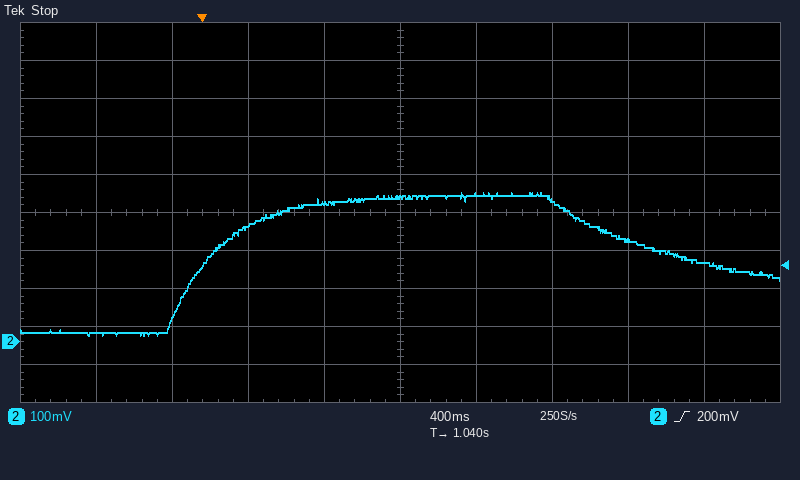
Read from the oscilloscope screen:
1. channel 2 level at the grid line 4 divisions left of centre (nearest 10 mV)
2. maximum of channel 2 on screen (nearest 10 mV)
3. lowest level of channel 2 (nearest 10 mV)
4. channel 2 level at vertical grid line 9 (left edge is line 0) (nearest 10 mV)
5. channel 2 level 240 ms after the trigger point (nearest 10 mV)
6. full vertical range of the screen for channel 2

20 mV
390 mV
20 mV
210 mV
300 mV
1 V
